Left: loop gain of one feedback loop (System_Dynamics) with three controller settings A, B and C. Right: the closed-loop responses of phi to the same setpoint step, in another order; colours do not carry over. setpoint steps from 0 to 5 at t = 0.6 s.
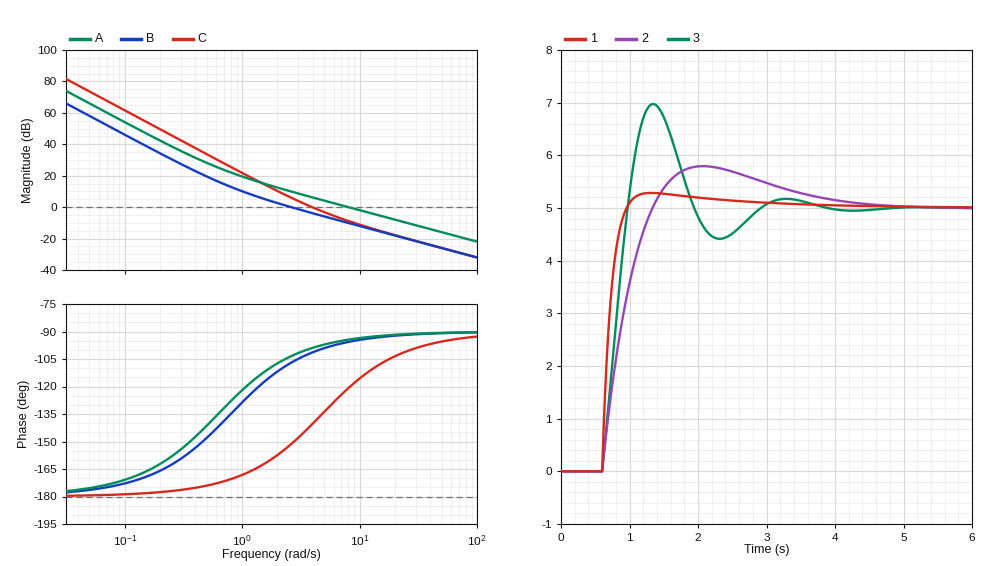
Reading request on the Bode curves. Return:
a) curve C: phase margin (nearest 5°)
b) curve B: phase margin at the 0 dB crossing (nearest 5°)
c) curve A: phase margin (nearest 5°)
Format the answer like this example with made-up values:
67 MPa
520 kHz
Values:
40°
75°
85°
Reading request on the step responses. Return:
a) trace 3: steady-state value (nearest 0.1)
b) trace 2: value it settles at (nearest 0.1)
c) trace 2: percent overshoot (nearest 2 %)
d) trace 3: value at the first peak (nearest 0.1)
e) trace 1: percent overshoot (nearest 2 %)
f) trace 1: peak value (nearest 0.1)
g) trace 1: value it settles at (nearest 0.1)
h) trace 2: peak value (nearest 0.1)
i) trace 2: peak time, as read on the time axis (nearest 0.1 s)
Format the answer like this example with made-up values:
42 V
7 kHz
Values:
5.0
5.0
16 %
7.0
6 %
5.3
5.0
5.8
2.1 s
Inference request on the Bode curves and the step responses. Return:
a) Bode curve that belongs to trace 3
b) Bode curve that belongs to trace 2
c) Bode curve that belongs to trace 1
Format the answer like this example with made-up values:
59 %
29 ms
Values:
C
B
A
